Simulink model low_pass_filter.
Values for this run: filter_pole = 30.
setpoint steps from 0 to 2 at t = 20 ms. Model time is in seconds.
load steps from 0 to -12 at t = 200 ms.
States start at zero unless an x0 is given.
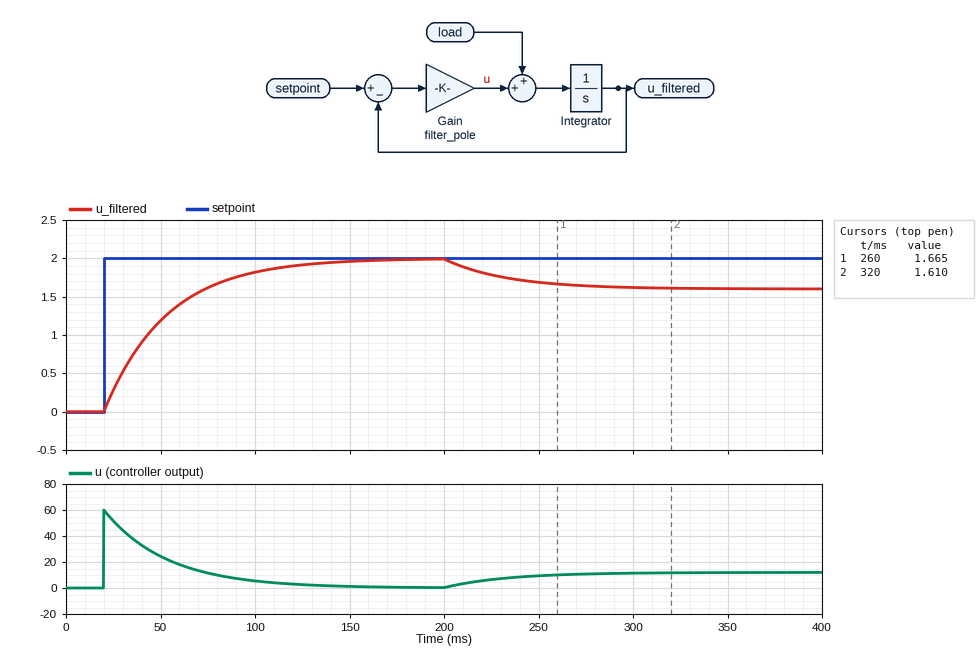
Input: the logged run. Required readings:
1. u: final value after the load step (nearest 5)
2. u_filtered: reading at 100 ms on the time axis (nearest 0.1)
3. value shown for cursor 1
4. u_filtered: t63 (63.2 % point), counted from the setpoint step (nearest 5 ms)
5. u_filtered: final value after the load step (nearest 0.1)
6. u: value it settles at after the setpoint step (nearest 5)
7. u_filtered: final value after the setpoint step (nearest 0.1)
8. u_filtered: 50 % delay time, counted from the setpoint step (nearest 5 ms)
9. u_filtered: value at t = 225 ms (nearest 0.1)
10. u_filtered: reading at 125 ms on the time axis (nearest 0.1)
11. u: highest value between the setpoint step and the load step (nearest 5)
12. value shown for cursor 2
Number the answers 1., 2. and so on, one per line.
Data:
1. 10
2. 1.8
3. 1.665
4. 35 ms
5. 1.6
6. 0
7. 2.0
8. 25 ms
9. 1.8
10. 1.9
11. 60
12. 1.610
